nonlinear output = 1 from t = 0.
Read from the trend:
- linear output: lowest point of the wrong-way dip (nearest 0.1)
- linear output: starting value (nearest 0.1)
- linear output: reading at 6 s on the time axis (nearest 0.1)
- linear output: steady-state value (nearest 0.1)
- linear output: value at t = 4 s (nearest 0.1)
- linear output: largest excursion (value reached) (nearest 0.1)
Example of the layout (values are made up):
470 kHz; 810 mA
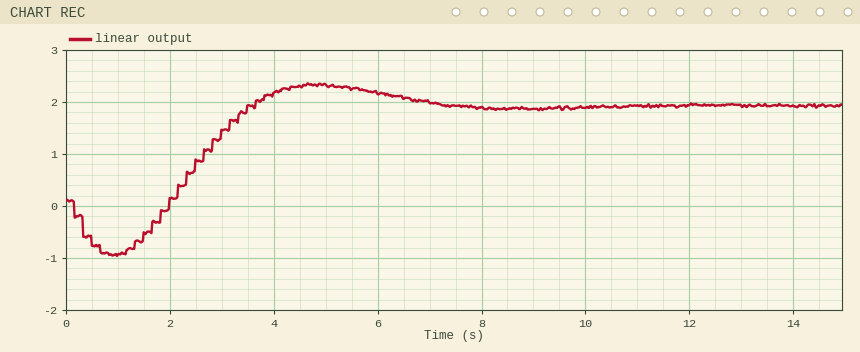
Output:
-0.9; 0.1; 2.2; 1.9; 2.2; 2.3
